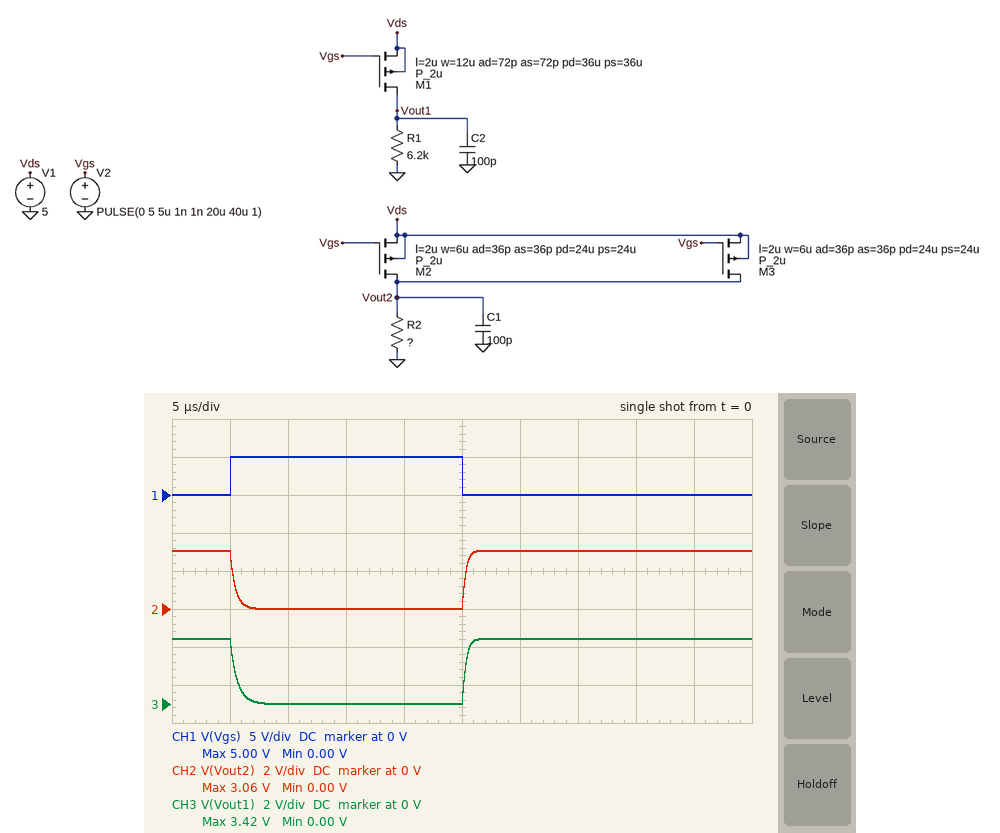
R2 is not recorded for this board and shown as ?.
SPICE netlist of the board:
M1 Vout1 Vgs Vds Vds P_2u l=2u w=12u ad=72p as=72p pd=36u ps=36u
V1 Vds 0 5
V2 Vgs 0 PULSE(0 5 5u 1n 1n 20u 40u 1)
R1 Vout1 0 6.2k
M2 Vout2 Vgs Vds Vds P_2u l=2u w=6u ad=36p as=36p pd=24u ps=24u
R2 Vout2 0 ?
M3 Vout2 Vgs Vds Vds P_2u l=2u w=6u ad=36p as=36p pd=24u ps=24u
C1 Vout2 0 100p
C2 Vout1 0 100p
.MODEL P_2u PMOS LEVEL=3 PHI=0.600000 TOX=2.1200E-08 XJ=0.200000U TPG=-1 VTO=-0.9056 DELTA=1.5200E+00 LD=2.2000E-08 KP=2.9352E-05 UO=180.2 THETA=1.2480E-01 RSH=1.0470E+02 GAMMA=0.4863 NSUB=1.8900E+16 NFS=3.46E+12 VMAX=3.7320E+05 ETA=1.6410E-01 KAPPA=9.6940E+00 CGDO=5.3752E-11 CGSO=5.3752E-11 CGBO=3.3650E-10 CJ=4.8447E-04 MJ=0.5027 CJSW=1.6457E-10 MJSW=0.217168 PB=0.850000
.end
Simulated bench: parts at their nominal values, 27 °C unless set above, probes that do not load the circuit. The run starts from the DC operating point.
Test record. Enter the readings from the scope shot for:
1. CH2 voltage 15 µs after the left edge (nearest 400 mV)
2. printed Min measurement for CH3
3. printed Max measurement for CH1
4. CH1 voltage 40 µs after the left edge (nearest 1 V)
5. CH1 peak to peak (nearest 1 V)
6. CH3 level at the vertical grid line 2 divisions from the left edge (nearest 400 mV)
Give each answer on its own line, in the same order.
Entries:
0 V
0.00 V
5.00 V
0 V
5 V
0 V
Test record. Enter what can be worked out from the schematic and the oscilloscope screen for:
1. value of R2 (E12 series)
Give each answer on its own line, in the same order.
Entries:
4.7 kΩ
